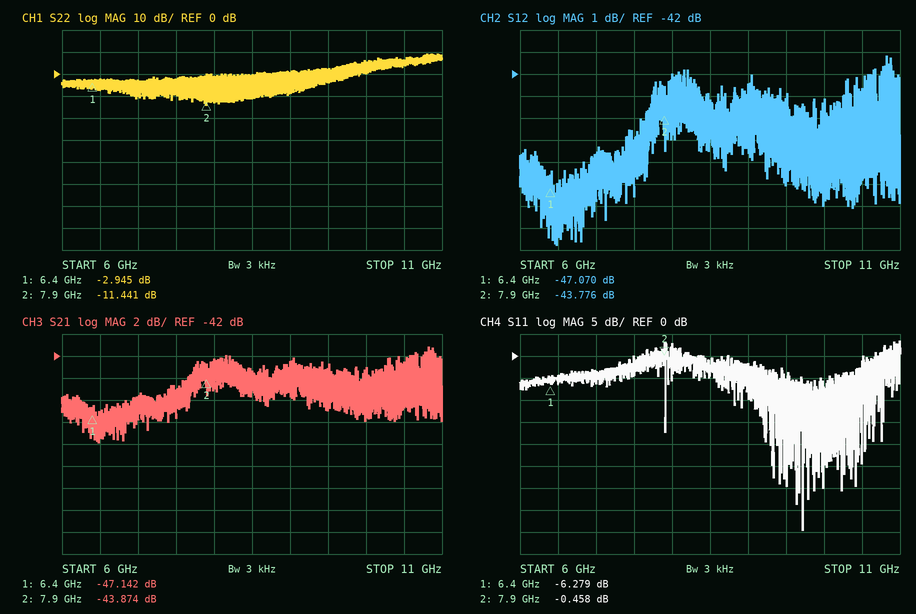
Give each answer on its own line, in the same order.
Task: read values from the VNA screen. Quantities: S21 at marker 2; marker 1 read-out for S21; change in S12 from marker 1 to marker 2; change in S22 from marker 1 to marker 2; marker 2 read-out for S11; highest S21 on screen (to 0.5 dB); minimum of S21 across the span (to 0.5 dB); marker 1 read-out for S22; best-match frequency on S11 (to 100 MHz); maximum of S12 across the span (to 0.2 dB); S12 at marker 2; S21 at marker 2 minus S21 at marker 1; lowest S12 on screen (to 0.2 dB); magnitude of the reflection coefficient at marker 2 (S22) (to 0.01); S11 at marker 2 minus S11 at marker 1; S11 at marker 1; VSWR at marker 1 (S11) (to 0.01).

-43.874 dB
-47.142 dB
3.294 dB
-8.496 dB
-0.458 dB
-41.0 dB
-50.0 dB
-2.945 dB
9.7 GHz
-41.2 dB
-43.776 dB
3.268 dB
-49.8 dB
0.27
5.821 dB
-6.279 dB
2.89
